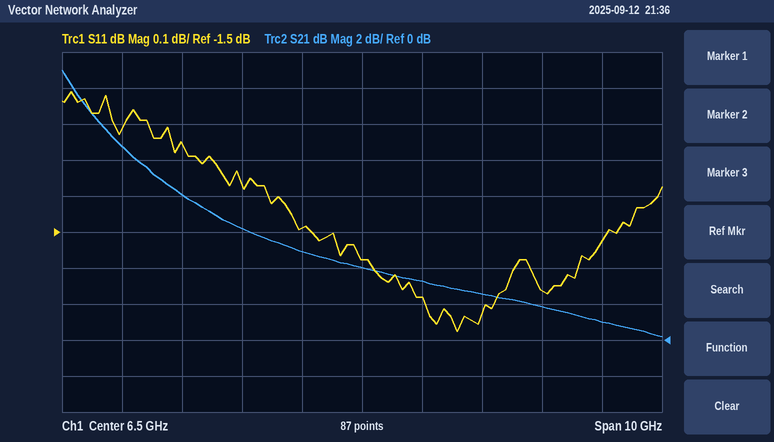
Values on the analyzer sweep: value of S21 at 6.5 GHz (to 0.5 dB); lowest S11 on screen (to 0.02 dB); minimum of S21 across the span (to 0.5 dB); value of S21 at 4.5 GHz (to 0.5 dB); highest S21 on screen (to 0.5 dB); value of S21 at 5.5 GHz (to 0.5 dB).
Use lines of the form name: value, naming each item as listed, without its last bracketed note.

value of S21 at 6.5 GHz: 4.0 dB
lowest S11 on screen: -1.78 dB
minimum of S21 across the span: 0.0 dB
value of S21 at 4.5 GHz: 6.0 dB
highest S21 on screen: 15.0 dB
value of S21 at 5.5 GHz: 5.0 dB
